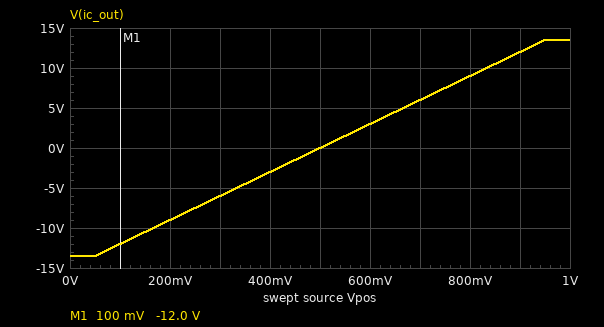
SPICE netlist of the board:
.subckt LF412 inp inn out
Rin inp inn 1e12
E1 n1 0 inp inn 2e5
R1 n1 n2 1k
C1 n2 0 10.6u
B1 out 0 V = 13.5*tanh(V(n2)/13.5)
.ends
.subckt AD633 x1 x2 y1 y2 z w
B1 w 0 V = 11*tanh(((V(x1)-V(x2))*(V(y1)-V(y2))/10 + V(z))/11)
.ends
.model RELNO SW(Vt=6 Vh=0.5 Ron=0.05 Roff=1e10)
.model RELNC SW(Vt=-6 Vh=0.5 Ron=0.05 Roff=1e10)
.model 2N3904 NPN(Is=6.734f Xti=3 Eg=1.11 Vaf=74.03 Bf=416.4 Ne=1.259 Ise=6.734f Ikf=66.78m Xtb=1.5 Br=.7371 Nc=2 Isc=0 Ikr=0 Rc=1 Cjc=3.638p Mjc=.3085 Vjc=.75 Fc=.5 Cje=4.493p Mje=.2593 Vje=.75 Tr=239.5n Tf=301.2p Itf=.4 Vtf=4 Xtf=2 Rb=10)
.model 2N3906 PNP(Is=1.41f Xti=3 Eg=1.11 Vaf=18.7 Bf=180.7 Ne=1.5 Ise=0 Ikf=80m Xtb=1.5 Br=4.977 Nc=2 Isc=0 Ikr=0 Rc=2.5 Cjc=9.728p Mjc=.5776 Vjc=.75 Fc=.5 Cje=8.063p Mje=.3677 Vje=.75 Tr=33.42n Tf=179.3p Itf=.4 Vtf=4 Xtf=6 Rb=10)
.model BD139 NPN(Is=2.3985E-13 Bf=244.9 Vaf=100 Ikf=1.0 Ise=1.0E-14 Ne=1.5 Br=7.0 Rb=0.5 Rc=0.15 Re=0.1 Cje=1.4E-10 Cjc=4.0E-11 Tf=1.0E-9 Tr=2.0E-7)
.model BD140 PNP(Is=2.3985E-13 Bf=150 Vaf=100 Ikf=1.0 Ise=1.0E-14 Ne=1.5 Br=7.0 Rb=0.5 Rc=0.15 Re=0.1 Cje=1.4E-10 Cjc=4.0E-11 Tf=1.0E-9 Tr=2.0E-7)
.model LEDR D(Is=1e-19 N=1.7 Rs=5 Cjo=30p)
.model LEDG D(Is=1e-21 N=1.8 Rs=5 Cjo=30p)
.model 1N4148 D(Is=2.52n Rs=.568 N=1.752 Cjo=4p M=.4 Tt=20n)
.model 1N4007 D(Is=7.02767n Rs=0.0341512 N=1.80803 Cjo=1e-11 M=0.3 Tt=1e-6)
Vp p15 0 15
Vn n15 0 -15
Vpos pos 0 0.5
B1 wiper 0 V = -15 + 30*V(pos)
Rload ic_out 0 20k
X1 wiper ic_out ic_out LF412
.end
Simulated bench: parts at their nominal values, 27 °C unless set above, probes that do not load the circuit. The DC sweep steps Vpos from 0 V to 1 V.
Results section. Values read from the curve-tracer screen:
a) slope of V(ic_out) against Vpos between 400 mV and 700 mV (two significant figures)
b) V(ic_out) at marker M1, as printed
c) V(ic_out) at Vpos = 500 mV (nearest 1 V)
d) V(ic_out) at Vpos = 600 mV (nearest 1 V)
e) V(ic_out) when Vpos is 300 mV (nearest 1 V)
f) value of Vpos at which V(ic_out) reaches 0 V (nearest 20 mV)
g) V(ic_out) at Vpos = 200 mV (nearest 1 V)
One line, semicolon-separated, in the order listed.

30 V/V; -12.0 V; 0 V; 3 V; -6 V; 500 mV; -9 V
